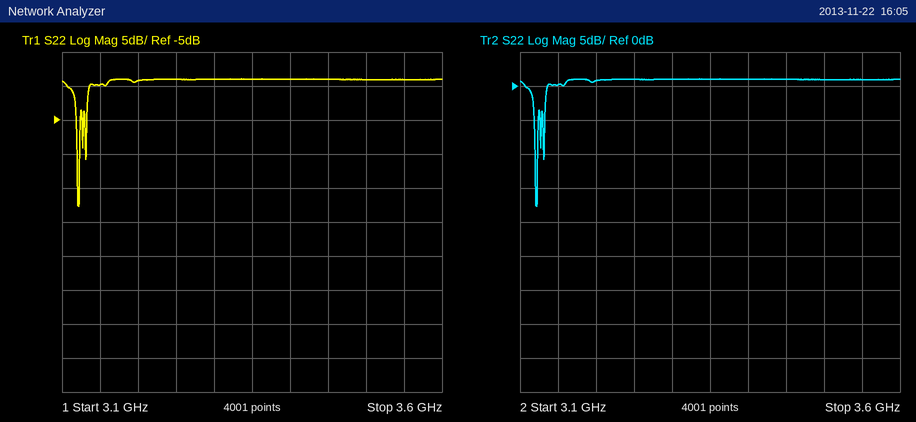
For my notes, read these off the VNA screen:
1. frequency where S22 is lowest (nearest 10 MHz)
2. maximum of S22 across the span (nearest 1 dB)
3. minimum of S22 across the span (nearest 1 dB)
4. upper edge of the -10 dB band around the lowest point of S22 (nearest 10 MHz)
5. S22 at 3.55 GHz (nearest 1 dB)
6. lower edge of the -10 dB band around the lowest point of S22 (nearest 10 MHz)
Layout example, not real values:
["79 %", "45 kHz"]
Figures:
["3.12 GHz", "1 dB", "-18 dB", "3.12 GHz", "1 dB", "3.12 GHz"]
